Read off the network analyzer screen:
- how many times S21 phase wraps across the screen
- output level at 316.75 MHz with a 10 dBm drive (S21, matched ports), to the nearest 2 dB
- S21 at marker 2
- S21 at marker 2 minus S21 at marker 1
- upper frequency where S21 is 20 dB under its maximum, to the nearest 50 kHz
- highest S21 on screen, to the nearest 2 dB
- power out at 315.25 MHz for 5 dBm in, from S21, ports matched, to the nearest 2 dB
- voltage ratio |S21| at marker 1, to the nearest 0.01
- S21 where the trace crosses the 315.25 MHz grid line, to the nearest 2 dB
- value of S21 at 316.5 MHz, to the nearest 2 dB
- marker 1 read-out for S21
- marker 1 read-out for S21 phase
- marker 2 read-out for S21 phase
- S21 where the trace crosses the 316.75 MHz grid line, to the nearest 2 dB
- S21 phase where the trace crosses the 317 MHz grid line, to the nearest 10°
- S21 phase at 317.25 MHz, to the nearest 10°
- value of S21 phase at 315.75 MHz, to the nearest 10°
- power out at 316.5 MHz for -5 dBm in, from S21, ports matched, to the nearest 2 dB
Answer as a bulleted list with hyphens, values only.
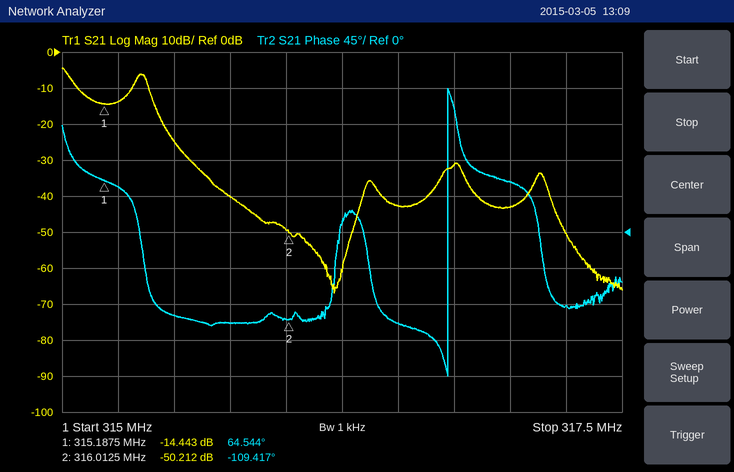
- 1
- -22 dBm
- -50.212 dB
- -35.769 dB
- 315.50 MHz
- -4 dB
- -8 dBm
- 0.19
- -14 dB
- -42 dB
- -14.443 dB
- 64.544°
- -109.417°
- -32 dB
- 60°
- -90°
- -110°
- -48 dBm
